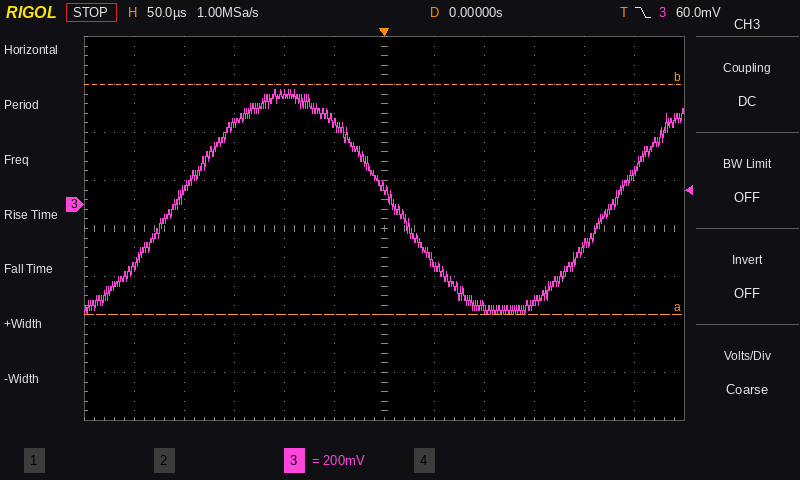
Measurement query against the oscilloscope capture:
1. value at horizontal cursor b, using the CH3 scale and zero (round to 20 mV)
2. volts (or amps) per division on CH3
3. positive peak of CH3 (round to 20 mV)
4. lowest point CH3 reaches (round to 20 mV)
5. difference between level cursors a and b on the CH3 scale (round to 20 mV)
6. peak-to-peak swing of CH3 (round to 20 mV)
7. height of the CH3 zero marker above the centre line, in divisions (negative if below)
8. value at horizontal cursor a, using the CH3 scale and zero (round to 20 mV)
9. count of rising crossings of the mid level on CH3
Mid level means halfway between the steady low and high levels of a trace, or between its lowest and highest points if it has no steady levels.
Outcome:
500 mV
200 mV
480 mV
-460 mV
960 mV
940 mV
+0.5 div
-460 mV
2
